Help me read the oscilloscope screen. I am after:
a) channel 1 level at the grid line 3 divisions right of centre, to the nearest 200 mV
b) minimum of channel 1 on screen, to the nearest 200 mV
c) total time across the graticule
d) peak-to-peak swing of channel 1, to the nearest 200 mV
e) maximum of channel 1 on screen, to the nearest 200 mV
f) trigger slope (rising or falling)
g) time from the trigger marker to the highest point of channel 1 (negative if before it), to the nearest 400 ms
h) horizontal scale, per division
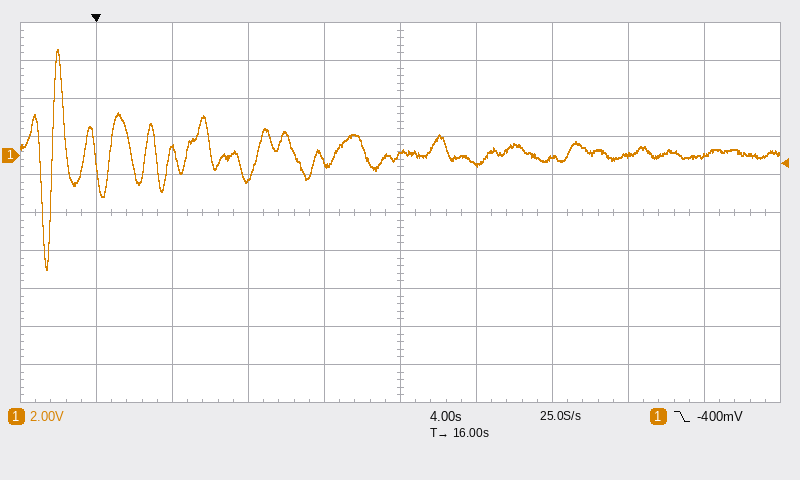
0.0 V
-6.0 V
40 s
11.6 V
5.6 V
falling
-2.0 s
4 s
